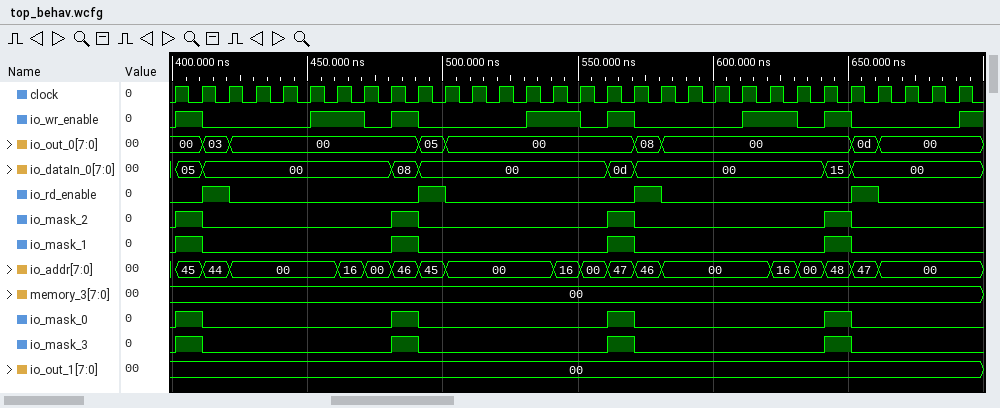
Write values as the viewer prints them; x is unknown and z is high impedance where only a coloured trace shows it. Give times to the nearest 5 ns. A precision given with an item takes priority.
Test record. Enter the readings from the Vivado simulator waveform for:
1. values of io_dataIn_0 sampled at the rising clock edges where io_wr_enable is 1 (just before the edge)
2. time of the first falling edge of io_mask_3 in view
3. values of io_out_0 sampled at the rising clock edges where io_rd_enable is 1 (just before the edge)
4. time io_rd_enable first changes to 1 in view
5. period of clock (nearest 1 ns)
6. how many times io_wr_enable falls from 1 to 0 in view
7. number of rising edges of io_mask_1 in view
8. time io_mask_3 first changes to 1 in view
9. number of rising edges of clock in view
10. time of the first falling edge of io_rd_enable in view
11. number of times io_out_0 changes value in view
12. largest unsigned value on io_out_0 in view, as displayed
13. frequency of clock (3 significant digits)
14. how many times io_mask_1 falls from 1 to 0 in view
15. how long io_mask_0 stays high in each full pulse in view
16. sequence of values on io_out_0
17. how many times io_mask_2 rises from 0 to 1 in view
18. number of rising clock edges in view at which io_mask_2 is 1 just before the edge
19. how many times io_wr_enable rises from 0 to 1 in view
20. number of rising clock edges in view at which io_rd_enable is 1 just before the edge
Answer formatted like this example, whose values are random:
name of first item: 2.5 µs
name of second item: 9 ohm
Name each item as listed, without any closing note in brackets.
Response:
values of io_dataIn_0 sampled at the rising clock edges where io_wr_enable is 1: 05, 00, 00, 08, 00, 00, 0d, 00, 00, 15
time of the first falling edge of io_mask_3 in view: 410 ns
values of io_out_0 sampled at the rising clock edges where io_rd_enable is 1: 03, 05, 08, 0d
time io_rd_enable first changes to 1 in view: 410 ns
period of clock: 10 ns
how many times io_wr_enable falls from 1 to 0 in view: 7
number of rising edges of io_mask_1 in view: 4
time io_mask_3 first changes to 1 in view: 400 ns
number of rising edges of clock in view: 30
time of the first falling edge of io_rd_enable in view: 420 ns
number of times io_out_0 changes value in view: 8
largest unsigned value on io_out_0 in view, as displayed: 0d
frequency of clock: 100 MHz
how many times io_mask_1 falls from 1 to 0 in view: 4
how long io_mask_0 stays high in each full pulse in view: 10 ns, 10 ns, 10 ns, 10 ns
sequence of values on io_out_0: 00, 03, 00, 05, 00, 08, 00, 0d, 00
how many times io_mask_2 rises from 0 to 1 in view: 4
number of rising clock edges in view at which io_mask_2 is 1 just before the edge: 4
how many times io_wr_enable rises from 0 to 1 in view: 8
number of rising clock edges in view at which io_rd_enable is 1 just before the edge: 4
